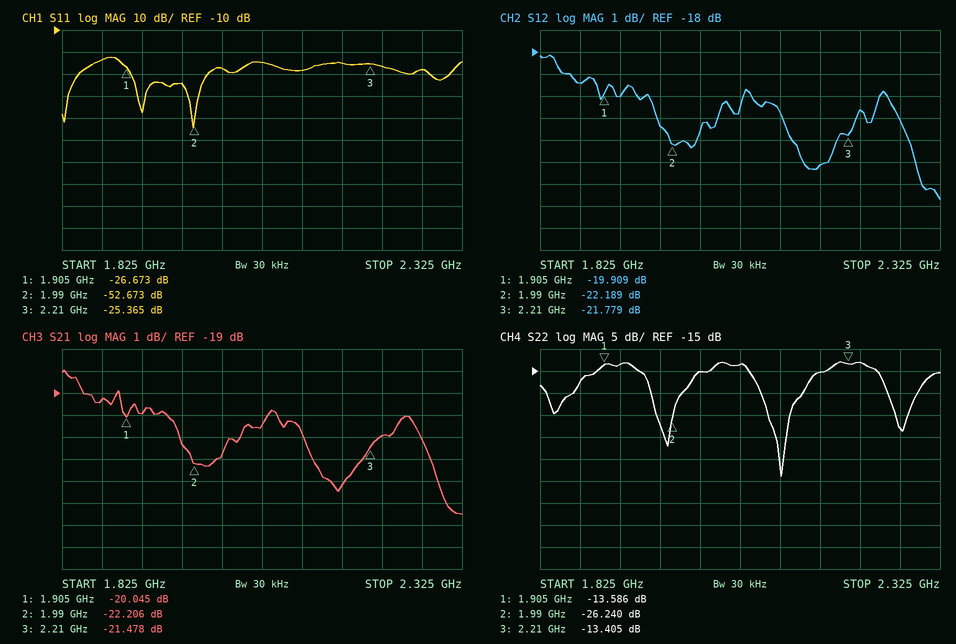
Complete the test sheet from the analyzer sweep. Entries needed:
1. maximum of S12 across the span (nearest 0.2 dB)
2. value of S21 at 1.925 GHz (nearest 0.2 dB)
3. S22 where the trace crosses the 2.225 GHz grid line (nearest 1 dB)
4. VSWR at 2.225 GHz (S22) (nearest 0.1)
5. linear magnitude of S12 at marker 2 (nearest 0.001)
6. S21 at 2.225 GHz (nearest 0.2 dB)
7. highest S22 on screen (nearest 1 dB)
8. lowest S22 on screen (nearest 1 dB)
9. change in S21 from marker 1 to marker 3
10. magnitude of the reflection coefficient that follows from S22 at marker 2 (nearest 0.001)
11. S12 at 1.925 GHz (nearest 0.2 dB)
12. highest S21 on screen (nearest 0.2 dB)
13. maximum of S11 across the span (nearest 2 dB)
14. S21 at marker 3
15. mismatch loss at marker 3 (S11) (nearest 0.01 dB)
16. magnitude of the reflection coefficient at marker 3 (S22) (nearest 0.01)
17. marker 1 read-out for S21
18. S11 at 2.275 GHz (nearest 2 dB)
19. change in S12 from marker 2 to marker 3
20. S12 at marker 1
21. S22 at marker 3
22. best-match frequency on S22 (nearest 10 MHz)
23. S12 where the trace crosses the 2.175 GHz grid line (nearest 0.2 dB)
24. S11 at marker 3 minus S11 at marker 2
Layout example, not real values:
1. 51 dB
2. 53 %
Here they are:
1. -18.2 dB
2. -20.0 dB
3. -13 dB
4. 1.6
5. 0.078
6. -21.0 dB
7. -13 dB
8. -39 dB
9. -1.433 dB
10. 0.049
11. -20.0 dB
12. -18.0 dB
13. -22 dB
14. -21.478 dB
15. 0.01 dB
16. 0.21
17. -20.045 dB
18. -28 dB
19. 0.410 dB
20. -19.909 dB
21. -13.405 dB
22. 2.13 GHz
23. -23.2 dB
24. 27.308 dB
